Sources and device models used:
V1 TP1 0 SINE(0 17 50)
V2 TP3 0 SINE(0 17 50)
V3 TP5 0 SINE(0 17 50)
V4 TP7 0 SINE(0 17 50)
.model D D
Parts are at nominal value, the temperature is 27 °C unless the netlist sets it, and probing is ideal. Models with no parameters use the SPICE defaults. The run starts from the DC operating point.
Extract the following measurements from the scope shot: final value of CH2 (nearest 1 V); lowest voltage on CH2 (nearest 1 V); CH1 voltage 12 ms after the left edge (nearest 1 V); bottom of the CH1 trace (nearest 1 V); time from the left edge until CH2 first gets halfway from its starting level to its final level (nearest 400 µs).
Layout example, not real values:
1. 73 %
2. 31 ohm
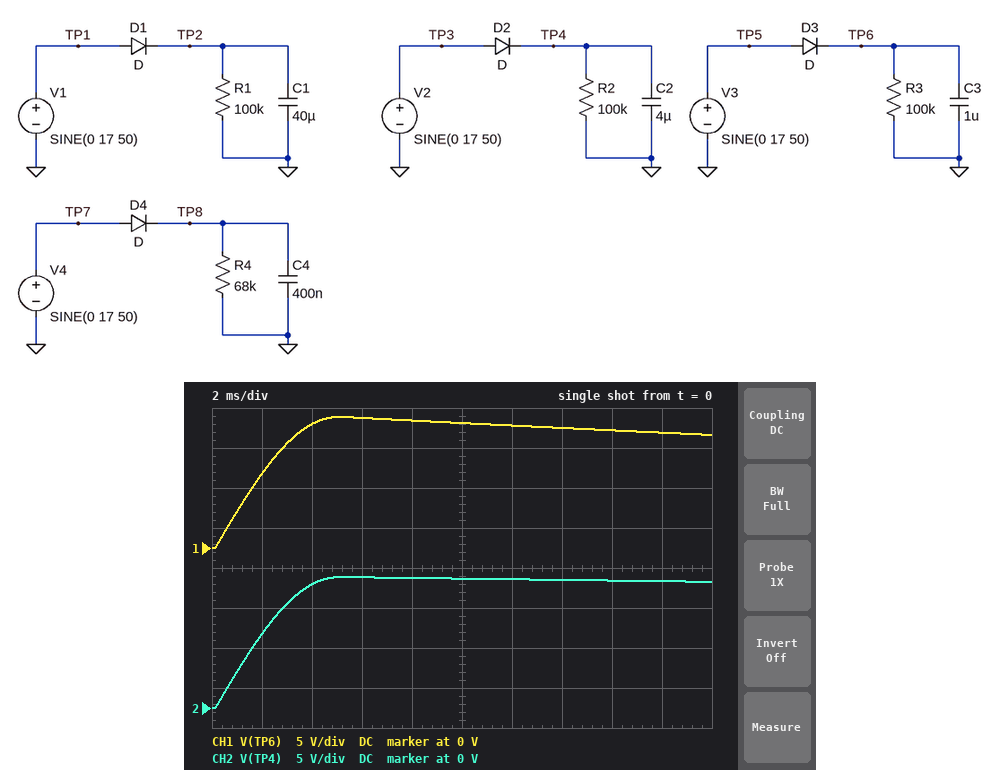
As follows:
1. 16 V
2. 0 V
3. 15 V
4. 0 V
5. 1.6 ms
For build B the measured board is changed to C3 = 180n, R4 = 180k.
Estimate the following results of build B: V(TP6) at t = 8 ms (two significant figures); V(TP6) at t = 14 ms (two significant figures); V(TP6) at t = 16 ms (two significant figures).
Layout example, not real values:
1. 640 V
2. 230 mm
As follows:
1. 14 V
2. 10 V
3. 9.1 V
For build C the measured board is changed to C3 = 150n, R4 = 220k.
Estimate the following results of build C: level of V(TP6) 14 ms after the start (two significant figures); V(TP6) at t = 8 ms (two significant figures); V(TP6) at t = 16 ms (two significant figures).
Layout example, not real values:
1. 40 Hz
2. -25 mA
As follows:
1. 9.2 V
2. 14 V
3. 8.1 V
